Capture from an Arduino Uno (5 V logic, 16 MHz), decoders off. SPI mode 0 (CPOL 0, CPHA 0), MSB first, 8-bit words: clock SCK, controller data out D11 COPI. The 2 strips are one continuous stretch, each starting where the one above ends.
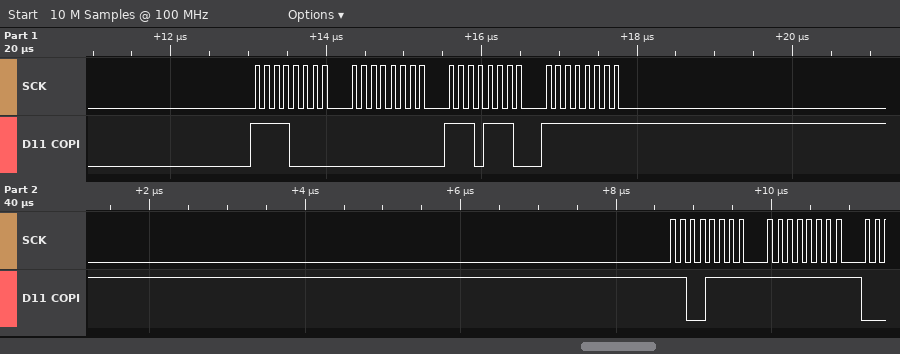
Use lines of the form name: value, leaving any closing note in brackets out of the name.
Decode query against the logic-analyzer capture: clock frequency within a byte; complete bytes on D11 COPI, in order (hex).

clock frequency within a byte: 8 MHz
complete bytes on D11 COPI, in order: 0xF0 0x00 0xEE 0xFF 0xCF 0xFF
